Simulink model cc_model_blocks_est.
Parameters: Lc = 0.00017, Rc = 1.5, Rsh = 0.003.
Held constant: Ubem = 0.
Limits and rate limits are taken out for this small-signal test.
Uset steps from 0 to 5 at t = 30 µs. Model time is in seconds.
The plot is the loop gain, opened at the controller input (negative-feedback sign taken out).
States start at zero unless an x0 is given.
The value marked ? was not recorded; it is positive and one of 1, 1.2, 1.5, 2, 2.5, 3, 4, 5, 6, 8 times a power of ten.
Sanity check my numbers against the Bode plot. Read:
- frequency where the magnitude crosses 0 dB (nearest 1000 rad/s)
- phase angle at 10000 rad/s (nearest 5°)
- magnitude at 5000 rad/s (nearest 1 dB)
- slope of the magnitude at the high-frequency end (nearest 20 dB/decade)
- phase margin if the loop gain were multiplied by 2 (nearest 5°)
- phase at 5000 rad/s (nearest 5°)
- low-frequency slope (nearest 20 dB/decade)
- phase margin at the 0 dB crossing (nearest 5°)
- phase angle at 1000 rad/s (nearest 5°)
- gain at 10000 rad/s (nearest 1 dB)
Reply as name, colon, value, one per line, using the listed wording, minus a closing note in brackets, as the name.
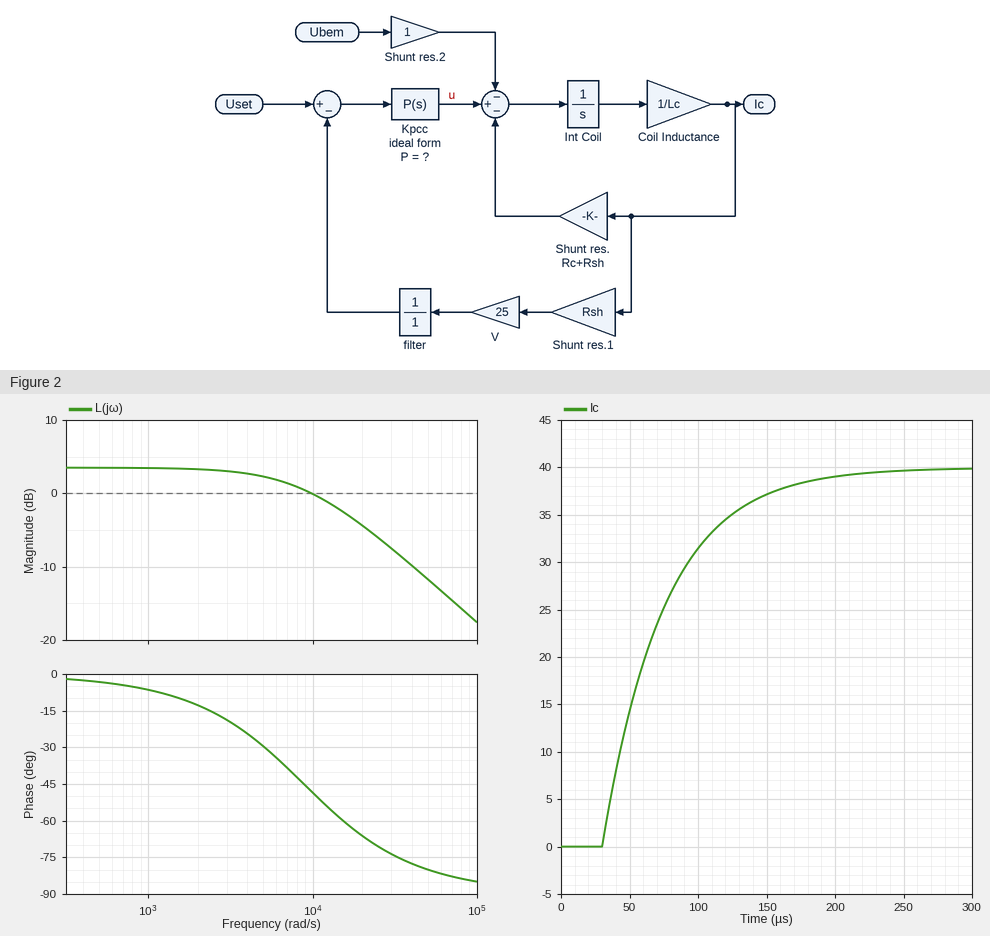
frequency where the magnitude crosses 0 dB: 10000 rad/s
phase angle at 10000 rad/s: -50°
magnitude at 5000 rad/s: 2 dB
slope of the magnitude at the high-frequency end: -20 dB/decade
phase margin if the loop gain were multiplied by 2: 110°
phase at 5000 rad/s: -30°
low-frequency slope: 0 dB/decade
phase margin at the 0 dB crossing: 130°
phase angle at 1000 rad/s: -5°
gain at 10000 rad/s: 0 dB
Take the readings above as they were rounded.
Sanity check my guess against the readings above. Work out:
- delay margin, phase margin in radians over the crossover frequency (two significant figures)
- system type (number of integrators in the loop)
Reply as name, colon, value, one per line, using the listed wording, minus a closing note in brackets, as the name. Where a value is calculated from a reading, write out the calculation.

delay margin, phase margin in radians over the crossover frequency: 130 × π / 180 / 10000 = 0.00023 s
system type: 0
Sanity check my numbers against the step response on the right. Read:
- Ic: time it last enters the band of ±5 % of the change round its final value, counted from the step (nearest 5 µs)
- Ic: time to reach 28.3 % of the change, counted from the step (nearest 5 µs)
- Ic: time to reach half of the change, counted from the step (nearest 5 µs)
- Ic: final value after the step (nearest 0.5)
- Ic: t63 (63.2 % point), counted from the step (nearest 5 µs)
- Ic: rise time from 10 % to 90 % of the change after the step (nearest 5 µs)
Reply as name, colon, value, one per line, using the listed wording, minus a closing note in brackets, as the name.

Ic: time it last enters the band of ±5 % of the change round its final value, counted from the step: 135 µs
Ic: time to reach 28.3 % of the change, counted from the step: 15 µs
Ic: time to reach half of the change, counted from the step: 30 µs
Ic: final value after the step: 40.0
Ic: t63 (63.2 % point), counted from the step: 45 µs
Ic: rise time from 10 % to 90 % of the change after the step: 100 µs
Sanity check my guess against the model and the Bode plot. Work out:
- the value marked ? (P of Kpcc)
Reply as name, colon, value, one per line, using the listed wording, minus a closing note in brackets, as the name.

the value marked ?: 30
